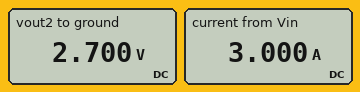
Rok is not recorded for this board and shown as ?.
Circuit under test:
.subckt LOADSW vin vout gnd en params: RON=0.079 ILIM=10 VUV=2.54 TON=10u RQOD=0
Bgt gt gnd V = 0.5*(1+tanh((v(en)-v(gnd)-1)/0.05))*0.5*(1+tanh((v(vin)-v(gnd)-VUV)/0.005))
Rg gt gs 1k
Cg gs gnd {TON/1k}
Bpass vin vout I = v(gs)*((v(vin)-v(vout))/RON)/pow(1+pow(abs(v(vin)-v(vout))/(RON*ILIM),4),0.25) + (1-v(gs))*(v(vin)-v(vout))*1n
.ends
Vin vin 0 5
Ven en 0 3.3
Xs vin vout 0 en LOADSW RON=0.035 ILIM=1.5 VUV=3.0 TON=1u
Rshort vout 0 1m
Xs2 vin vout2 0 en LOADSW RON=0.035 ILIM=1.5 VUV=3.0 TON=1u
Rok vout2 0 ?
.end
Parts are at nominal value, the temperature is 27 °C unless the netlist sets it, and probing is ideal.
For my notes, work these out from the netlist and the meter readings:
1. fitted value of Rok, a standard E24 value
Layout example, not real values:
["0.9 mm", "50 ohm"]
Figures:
["1.8 Ω"]
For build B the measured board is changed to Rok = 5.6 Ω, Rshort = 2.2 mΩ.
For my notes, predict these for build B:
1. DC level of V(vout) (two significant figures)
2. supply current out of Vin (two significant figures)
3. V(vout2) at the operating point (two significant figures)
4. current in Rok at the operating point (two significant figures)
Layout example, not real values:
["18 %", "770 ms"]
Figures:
["3.3 mV", "2.4 A", "5.0 V", "890 mA"]
